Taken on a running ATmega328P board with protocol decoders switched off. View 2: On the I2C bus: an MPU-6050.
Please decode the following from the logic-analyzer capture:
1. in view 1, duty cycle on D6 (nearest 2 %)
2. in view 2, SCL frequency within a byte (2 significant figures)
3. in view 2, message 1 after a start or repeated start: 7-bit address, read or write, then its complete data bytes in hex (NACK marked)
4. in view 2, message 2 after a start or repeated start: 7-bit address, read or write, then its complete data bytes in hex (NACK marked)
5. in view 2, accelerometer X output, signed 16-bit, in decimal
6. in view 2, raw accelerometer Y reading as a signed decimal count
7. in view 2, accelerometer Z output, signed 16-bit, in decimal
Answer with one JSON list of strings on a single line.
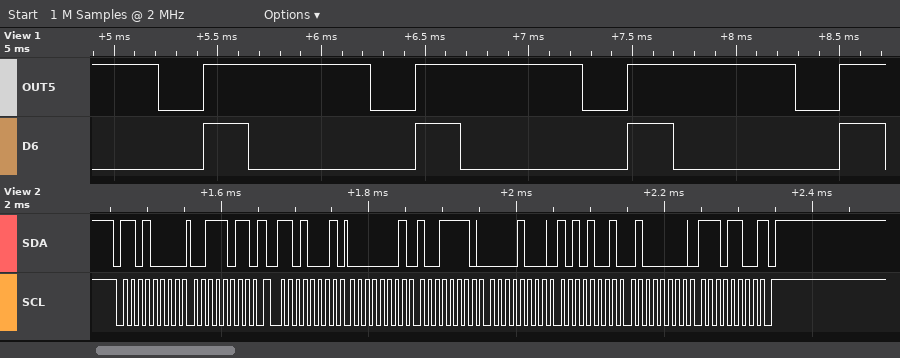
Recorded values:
["22 %", "100 kHz", "0x68 write: 3B", "0x68 read: 01 9E 08 A9 40 EC NACK", "414", "2217", "16620"]
